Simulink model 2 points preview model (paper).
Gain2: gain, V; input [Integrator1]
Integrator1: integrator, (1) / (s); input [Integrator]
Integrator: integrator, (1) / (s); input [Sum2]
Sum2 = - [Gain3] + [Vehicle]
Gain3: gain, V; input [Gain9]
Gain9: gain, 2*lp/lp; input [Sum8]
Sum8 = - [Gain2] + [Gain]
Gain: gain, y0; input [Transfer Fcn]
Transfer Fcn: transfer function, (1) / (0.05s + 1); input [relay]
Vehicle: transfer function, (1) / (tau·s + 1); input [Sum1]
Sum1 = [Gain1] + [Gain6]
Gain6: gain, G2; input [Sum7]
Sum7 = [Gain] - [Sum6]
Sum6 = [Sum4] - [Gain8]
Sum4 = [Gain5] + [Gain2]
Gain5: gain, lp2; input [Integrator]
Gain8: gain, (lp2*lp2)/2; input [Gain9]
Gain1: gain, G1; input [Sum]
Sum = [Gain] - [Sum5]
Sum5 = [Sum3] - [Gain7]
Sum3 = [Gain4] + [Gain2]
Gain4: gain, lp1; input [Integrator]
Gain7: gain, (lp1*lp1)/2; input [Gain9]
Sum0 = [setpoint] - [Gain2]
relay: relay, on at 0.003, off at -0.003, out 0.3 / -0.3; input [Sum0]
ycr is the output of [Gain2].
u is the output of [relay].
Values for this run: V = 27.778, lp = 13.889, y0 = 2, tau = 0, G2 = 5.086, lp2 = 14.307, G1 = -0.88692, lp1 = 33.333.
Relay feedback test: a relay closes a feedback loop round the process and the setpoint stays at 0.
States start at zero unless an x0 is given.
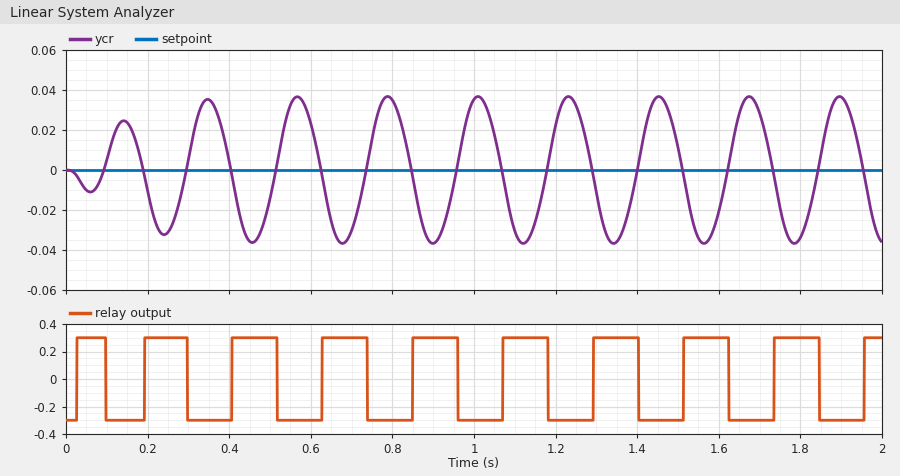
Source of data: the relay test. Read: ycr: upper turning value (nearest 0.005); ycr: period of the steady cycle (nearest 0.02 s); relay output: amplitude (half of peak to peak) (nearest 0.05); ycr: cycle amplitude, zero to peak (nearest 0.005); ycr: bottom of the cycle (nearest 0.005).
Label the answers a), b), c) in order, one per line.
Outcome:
a) 0.035
b) 0.22 s
c) 0.30
d) 0.035
e) -0.035
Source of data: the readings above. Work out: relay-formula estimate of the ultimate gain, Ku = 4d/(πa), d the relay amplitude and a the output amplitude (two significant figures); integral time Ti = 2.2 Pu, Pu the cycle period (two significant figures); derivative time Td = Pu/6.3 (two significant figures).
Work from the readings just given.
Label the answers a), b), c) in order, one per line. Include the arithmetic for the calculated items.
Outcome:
a) 4 × 0.3 / (π × 0.035) = 11
b) 2.2 × 0.22 = 0.48 s
c) 0.22 / 6.3 = 0.035 s
